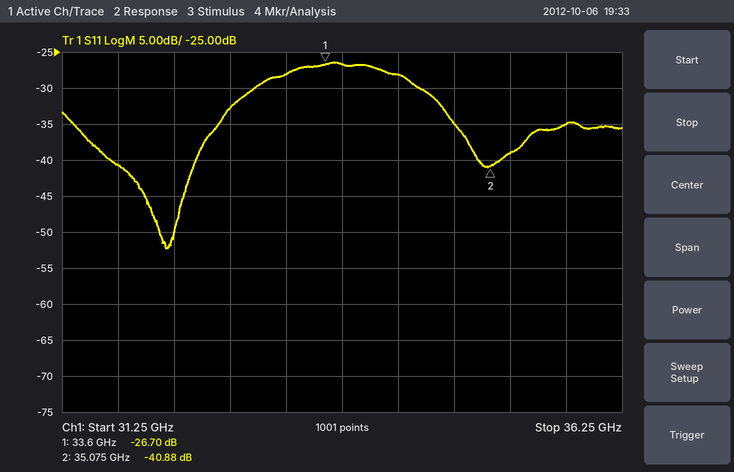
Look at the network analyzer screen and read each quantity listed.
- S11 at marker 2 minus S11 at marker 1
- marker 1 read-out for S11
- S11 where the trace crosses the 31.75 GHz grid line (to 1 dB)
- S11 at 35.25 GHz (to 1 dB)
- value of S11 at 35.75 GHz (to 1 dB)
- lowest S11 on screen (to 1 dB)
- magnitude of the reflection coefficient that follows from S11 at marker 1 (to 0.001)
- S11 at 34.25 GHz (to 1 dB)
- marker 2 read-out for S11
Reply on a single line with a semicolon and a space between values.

-14.18 dB; -26.70 dB; -41 dB; -39 dB; -35 dB; -52 dB; 0.046; -28 dB; -40.88 dB
